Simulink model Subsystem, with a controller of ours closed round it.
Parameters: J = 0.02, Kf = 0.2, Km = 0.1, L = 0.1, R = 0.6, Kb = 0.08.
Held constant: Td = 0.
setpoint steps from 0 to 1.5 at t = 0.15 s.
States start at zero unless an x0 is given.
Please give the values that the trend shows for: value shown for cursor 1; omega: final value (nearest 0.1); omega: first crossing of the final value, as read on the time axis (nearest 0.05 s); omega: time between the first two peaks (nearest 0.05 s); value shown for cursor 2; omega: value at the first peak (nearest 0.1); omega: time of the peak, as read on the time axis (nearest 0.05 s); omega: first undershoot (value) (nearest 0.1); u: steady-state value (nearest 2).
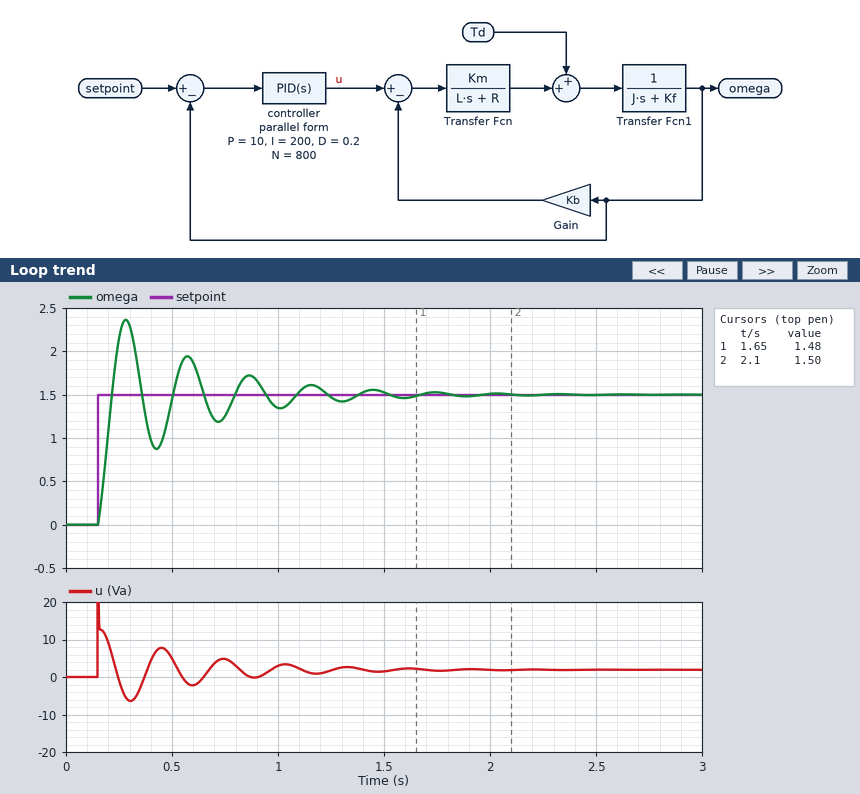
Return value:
1.48
1.5
0.20 s
0.30 s
1.50
2.4
0.30 s
0.9
2
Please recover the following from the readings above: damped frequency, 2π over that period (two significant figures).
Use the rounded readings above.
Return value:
21 rad/s
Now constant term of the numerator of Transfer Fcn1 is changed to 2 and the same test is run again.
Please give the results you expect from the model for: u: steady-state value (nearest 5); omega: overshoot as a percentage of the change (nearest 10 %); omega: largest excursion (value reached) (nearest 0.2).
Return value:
0
50 %
2.2
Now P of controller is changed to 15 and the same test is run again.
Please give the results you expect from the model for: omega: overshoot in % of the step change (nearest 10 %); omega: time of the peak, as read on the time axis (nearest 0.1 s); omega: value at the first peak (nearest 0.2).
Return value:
50 %
0.3 s
2.2
